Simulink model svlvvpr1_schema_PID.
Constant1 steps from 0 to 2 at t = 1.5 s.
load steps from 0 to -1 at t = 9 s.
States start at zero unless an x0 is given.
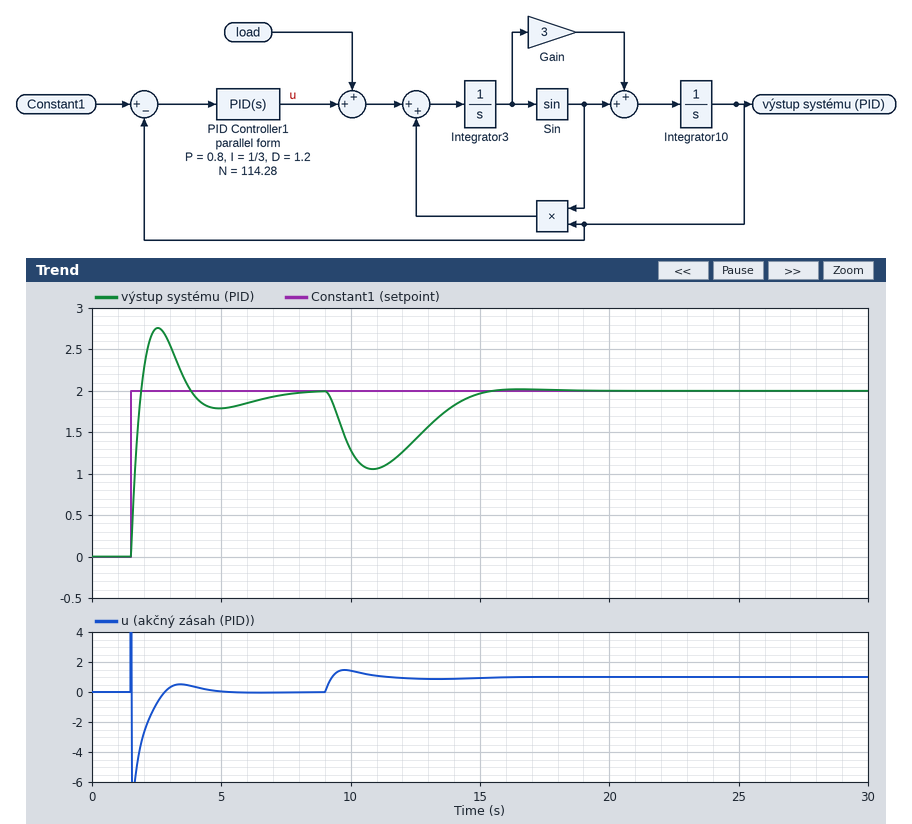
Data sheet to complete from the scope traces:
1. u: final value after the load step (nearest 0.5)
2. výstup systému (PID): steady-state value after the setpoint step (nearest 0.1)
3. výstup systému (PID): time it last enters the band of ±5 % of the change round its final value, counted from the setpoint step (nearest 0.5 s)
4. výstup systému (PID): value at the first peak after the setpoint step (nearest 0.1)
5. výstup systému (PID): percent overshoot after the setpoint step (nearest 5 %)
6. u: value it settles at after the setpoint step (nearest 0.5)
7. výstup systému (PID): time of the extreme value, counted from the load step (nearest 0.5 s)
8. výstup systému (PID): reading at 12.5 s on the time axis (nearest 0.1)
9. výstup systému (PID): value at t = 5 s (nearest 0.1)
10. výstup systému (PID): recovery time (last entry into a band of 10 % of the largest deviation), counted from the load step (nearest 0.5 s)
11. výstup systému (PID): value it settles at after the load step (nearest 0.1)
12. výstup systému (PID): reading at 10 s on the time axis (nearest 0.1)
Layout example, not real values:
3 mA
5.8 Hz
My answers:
1.0
2.0
5.0 s
2.8
40 %
0.0
2.0 s
1.4
1.8
5.5 s
2.0
1.3
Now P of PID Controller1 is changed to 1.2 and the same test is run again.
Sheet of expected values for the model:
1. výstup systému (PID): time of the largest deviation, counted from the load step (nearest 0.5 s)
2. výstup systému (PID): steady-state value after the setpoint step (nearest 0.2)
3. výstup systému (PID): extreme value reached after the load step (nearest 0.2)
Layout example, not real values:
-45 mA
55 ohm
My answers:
1.5 s
2.0
1.2
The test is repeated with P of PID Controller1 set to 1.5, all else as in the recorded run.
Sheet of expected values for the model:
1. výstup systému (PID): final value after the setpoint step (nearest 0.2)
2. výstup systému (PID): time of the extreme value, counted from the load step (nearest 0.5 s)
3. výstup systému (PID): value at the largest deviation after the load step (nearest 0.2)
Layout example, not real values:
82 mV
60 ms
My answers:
2.0
1.5 s
1.4
